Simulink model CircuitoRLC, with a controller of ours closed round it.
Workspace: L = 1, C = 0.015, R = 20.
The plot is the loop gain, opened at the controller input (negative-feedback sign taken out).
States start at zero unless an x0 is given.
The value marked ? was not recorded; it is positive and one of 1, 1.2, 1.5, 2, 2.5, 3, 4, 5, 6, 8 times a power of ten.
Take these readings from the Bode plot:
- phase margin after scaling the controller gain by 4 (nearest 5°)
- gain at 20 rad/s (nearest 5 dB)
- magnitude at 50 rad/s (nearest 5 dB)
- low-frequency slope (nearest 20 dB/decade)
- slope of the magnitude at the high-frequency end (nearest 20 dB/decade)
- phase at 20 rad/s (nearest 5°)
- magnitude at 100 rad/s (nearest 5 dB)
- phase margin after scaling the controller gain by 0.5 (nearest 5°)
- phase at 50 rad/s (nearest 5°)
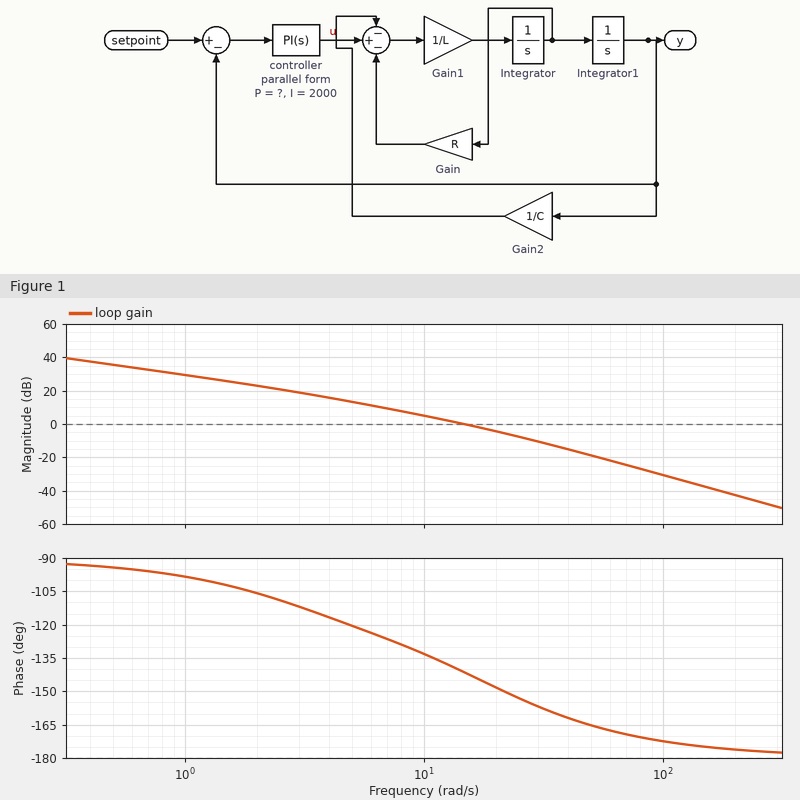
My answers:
20°
-5 dB
-20 dB
-20 dB/decade
-40 dB/decade
-150°
-30 dB
50°
-165°
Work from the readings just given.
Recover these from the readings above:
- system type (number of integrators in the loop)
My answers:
1
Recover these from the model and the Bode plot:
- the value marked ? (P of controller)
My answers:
300
